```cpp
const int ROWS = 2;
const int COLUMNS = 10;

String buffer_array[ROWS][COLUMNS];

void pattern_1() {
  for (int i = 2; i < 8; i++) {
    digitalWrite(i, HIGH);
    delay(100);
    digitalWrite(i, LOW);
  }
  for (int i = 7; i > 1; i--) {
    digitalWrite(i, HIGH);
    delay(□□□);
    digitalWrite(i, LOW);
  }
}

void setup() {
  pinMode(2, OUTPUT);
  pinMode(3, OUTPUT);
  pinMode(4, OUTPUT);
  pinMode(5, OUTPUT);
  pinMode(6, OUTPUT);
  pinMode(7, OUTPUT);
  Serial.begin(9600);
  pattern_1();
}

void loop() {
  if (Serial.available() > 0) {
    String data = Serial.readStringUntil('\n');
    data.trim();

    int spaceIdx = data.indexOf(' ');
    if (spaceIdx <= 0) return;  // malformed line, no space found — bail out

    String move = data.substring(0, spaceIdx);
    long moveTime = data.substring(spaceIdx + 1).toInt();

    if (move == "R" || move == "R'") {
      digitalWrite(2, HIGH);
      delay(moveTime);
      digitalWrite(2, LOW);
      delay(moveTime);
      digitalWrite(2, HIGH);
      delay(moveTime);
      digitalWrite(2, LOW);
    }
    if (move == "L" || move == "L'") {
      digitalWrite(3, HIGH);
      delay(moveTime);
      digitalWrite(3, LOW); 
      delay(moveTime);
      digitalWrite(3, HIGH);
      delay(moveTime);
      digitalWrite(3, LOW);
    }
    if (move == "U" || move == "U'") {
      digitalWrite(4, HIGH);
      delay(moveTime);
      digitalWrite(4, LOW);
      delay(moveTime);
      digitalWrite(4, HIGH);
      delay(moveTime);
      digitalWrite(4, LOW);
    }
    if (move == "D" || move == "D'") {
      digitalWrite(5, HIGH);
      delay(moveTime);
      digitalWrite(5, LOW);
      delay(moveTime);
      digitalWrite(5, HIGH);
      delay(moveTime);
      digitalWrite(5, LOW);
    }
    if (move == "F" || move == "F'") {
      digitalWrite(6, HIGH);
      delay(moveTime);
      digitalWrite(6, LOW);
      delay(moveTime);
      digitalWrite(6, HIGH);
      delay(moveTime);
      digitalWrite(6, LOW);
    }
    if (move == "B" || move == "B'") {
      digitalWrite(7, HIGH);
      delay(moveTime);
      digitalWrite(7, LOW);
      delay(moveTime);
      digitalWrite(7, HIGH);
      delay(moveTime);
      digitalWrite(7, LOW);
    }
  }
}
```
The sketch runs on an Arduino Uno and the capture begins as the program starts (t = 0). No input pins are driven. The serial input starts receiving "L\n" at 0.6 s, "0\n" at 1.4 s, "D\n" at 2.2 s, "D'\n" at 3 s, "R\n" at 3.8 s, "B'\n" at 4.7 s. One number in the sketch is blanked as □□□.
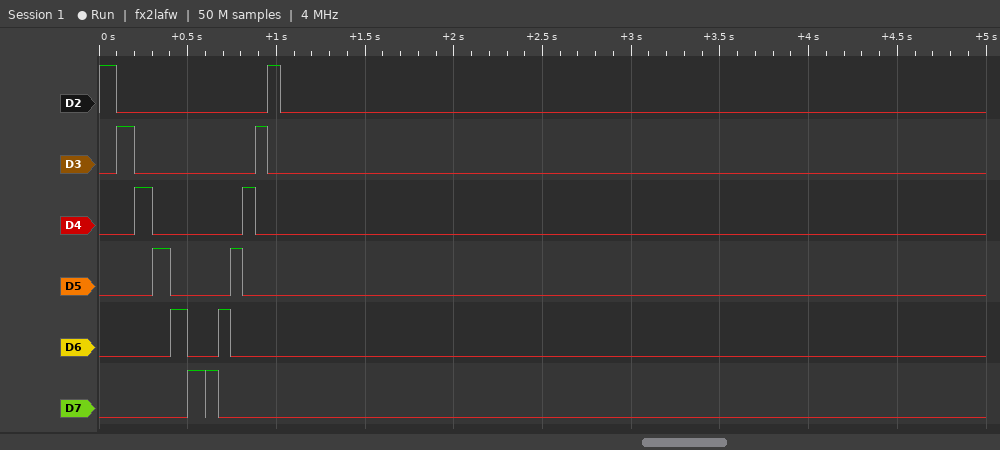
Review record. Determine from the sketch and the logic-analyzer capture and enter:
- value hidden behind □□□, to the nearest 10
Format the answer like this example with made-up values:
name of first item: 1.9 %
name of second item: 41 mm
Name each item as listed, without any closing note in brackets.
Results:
value hidden behind □□□, to the nearest 10: 70
